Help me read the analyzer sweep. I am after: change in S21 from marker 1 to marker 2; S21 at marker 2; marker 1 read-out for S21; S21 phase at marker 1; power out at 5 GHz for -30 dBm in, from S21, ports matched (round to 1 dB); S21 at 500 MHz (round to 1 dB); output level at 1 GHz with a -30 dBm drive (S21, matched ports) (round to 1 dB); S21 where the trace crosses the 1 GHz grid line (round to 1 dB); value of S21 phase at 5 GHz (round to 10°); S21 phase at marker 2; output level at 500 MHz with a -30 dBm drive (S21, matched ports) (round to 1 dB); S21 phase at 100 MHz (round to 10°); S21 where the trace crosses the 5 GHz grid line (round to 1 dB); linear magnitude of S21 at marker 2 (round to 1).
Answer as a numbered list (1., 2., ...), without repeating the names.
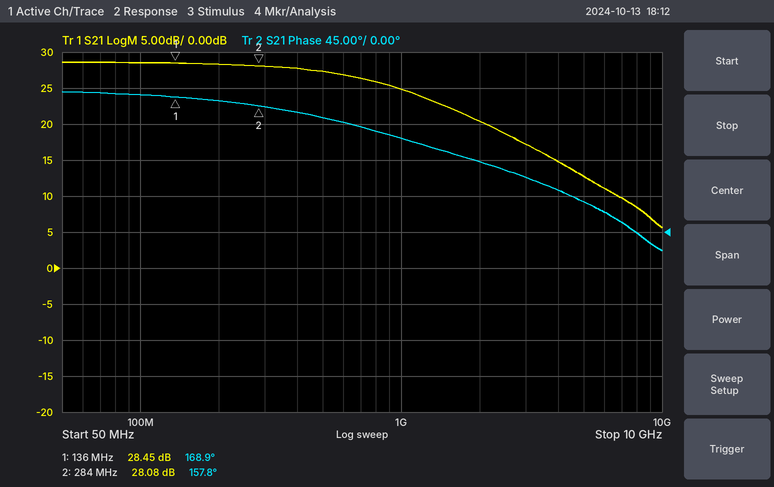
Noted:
1. -0.37 dB
2. 28.08 dB
3. 28.45 dB
4. 168.9°
5. -17 dBm
6. 27 dB
7. -5 dBm
8. 25 dB
9. 40°
10. 157.8°
11. -3 dBm
12. 170°
13. 13 dB
14. 25
